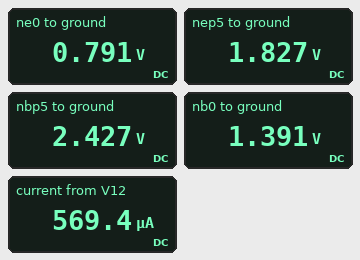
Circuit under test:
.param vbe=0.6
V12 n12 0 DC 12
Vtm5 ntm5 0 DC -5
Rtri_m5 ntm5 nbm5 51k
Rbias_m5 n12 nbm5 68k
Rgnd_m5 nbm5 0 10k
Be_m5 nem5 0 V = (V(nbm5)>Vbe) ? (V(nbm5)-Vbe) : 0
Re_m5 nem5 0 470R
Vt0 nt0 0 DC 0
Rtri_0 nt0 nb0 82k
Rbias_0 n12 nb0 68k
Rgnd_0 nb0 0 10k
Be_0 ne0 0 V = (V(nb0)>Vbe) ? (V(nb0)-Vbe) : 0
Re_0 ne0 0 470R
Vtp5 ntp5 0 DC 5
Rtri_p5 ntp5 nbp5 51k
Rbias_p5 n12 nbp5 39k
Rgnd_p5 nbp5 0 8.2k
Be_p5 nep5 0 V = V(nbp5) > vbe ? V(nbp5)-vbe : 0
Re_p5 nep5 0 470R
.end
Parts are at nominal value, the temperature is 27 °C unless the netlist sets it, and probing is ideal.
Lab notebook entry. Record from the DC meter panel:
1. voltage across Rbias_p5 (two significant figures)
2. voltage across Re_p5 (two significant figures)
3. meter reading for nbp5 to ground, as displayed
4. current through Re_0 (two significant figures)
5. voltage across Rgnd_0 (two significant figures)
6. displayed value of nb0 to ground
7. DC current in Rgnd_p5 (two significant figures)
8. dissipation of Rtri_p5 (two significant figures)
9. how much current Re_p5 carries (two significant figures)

9.6 V
1.8 V
2.427 V
1.7 mA
1.4 V
1.391 V
300 µA
130 µW
3.9 mA
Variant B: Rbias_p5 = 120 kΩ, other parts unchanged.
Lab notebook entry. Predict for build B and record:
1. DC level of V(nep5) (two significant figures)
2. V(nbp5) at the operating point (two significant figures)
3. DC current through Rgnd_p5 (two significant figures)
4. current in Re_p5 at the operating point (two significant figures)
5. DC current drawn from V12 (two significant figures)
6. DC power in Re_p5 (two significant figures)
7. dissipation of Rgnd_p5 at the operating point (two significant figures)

720 mV
1.3 V
160 µA
1.5 mA
410 µA
1.1 mW
210 µW
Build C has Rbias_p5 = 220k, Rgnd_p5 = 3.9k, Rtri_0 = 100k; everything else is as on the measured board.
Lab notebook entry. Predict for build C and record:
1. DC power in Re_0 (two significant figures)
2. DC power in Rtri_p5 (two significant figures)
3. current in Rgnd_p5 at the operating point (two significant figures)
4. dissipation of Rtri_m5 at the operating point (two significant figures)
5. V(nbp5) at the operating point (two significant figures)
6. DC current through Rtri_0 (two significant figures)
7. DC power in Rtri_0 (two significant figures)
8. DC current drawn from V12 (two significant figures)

1.4 mW
390 µW
140 µA
610 µW
540 mV
14 µA
20 µW
380 µA
